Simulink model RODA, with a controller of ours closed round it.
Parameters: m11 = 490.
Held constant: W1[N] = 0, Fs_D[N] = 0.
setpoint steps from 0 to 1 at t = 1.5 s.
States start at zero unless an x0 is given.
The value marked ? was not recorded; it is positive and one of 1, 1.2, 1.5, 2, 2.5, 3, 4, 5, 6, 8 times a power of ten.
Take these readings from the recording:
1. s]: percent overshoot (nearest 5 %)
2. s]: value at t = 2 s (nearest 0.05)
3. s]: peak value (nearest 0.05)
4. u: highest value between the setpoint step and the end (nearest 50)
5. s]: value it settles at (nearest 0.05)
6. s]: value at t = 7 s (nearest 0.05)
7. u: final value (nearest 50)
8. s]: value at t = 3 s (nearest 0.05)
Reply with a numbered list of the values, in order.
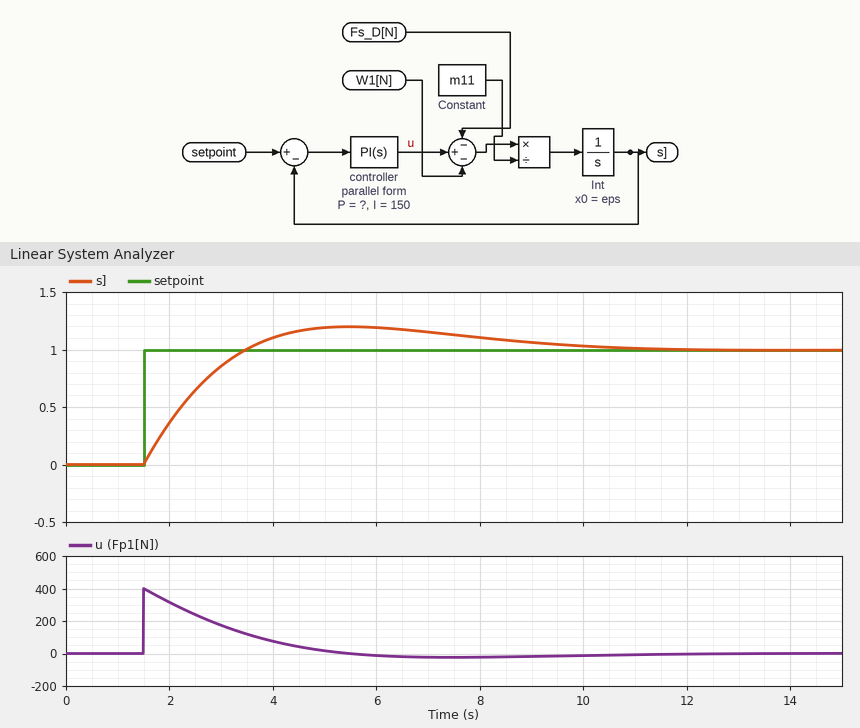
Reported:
1. 20 %
2. 0.35
3. 1.20
4. 400
5. 1.00
6. 1.15
7. 0
8. 0.85
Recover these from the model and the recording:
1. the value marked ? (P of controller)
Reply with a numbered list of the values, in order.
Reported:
1. 400
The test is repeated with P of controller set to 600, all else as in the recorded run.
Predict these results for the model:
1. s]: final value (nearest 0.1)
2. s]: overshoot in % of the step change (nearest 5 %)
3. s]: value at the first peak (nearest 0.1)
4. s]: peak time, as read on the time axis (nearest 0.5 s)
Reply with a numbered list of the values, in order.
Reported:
1. 1.0
2. 10 %
3. 1.1
4. 5.0 s
